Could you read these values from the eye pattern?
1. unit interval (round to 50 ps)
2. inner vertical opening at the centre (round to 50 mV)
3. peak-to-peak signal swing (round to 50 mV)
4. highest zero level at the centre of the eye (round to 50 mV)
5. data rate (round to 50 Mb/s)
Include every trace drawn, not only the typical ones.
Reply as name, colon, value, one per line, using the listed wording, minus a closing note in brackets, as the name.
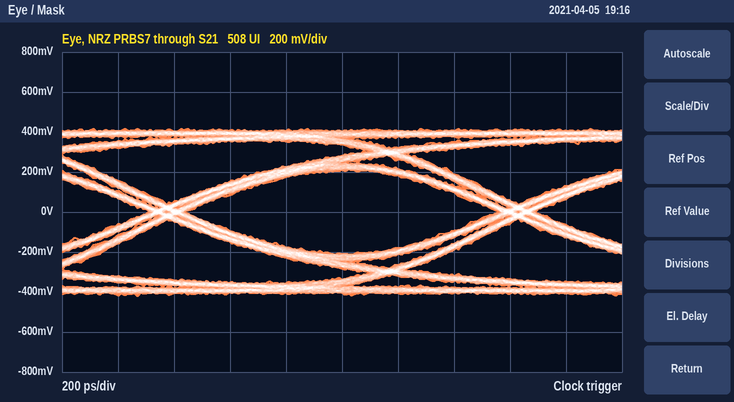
unit interval: 1.25 ns
inner vertical opening at the centre: 400 mV
peak-to-peak signal swing: 850 mV
highest zero level at the centre of the eye: -200 mV
data rate: 800 Mb/s
